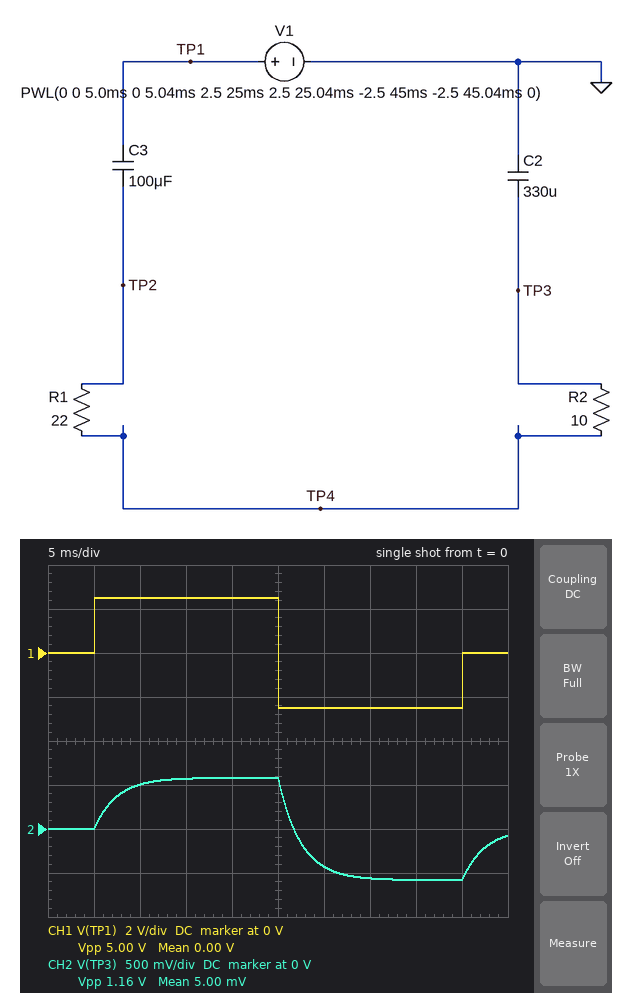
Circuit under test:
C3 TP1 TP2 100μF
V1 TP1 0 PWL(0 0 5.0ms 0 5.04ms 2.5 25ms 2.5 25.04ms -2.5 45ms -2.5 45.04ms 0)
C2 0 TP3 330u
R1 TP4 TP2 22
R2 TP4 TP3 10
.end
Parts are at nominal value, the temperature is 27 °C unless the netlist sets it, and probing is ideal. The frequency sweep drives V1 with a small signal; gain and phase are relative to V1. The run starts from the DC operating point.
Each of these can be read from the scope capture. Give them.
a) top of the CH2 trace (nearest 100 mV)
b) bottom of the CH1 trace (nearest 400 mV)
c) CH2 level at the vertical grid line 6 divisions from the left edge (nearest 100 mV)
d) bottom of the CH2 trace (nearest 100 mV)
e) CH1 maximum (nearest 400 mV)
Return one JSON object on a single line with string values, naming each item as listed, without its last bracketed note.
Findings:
{"top of the CH2 trace": "600 mV", "bottom of the CH1 trace": "-2.4 V", "CH2 level at the vertical grid line 6 divisions from the left edge": "-400 mV", "bottom of the CH2 trace": "-600 mV", "CH1 maximum": "2.4 V"}
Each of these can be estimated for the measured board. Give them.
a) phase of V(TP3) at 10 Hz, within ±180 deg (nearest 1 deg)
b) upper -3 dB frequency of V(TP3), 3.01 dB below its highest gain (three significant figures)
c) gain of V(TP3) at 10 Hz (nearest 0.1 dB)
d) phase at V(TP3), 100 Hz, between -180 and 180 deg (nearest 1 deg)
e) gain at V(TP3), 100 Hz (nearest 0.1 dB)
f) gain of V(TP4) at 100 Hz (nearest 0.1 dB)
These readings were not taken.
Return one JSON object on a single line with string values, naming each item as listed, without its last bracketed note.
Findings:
{"phase of V(TP3) at 10 Hz, within ±180 deg": "-9 deg", "upper -3 dB frequency of V(TP3), 3.01 dB below its highest gain": "64.8 Hz", "gain of V(TP3) at 10 Hz": "-12.8 dB", "phase at V(TP3), 100 Hz, between -180 and 180 deg": "-57 deg", "gain at V(TP3), 100 Hz": "-18.0 dB", "gain of V(TP4) at 100 Hz": "-10.7 dB"}
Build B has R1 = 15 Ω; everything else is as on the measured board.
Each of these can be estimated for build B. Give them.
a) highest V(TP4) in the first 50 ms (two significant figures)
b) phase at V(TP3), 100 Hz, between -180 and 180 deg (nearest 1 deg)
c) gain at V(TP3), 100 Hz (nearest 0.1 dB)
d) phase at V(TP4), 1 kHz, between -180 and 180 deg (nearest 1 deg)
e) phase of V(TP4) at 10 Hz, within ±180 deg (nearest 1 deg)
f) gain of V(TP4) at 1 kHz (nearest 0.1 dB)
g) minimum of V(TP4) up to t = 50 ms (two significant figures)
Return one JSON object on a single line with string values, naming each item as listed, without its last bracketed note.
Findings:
{"highest V(TP4) in the first 50 ms": "1.0 V", "phase at V(TP3), 100 Hz, between -180 and 180 deg": "-50 deg", "gain at V(TP3), 100 Hz": "-16.6 dB", "phase at V(TP4), 1 kHz, between -180 and 180 deg": "2 deg", "phase of V(TP4) at 10 Hz, within ±180 deg": "5 deg", "gain of V(TP4) at 1 kHz": "-8.0 dB", "minimum of V(TP4) up to t = 50 ms": "-1.4 V"}
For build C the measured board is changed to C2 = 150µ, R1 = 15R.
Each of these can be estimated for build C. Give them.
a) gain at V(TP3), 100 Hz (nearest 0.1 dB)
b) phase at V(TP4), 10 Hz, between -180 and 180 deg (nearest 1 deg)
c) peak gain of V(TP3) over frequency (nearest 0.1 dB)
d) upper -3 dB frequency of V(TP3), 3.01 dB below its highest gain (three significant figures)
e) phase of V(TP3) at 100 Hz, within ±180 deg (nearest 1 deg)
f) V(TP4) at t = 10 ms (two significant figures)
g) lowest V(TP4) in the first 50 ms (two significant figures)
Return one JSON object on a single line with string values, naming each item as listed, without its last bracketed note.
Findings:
{"gain at V(TP3), 100 Hz": "-10.7 dB", "phase at V(TP4), 10 Hz, between -180 and 180 deg": "0 deg", "peak gain of V(TP3) over frequency": "-8.0 dB", "upper -3 dB frequency of V(TP3), 3.01 dB below its highest gain": "106 Hz", "phase of V(TP3) at 100 Hz, within ±180 deg": "-43 deg", "V(TP4) at t = 10 ms": "1.0 V", "lowest V(TP4) in the first 50 ms": "-1.0 V"}
